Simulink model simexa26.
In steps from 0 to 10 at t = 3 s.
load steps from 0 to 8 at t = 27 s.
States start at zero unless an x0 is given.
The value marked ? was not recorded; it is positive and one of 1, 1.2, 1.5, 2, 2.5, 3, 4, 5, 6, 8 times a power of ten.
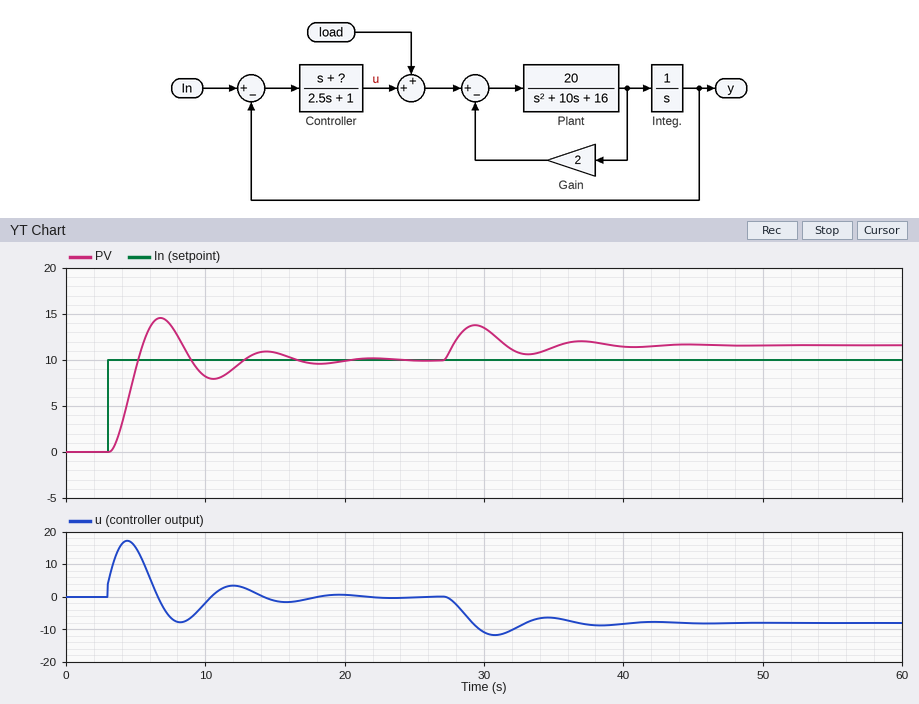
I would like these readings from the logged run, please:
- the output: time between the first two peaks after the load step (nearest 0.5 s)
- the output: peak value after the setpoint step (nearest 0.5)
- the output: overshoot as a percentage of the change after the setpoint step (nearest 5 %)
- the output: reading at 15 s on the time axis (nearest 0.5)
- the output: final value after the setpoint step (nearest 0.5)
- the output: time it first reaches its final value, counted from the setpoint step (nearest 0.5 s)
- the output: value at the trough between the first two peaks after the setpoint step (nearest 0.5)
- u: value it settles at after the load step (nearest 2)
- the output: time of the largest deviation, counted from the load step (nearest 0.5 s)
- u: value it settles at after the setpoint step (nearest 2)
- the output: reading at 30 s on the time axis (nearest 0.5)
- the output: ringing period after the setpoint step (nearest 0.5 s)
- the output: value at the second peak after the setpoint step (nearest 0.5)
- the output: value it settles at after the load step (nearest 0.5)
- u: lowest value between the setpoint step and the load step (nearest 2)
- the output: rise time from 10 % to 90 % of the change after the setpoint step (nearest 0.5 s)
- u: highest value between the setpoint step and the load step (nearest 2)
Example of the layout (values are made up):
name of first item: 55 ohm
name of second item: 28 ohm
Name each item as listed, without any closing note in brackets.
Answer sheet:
the output: time between the first two peaks after the load step: 7.5 s
the output: peak value after the setpoint step: 14.5
the output: overshoot as a percentage of the change after the setpoint step: 45 %
the output: reading at 15 s on the time axis: 11.0
the output: final value after the setpoint step: 10.0
the output: time it first reaches its final value, counted from the setpoint step: 2.0 s
the output: value at the trough between the first two peaks after the setpoint step: 8.0
u: value it settles at after the load step: -8
the output: time of the largest deviation, counted from the load step: 2.5 s
u: value it settles at after the setpoint step: 0
the output: reading at 30 s on the time axis: 13.5
the output: ringing period after the setpoint step: 7.5 s
the output: value at the second peak after the setpoint step: 11.0
the output: value it settles at after the load step: 11.5
u: lowest value between the setpoint step and the load step: -8
the output: rise time from 10 % to 90 % of the change after the setpoint step: 1.5 s
u: highest value between the setpoint step and the load step: 18
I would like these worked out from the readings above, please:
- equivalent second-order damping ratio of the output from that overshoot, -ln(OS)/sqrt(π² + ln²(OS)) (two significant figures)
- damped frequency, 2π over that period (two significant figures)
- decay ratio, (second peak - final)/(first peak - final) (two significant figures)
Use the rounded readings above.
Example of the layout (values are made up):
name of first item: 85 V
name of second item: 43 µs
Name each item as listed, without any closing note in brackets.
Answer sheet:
equivalent second-order damping ratio of the output from that overshoot, -ln(OS)/sqrt(π² + ln²(OS)): 0.25
damped frequency, 2π over that period: 0.84 rad/s
decay ratio, (second peak - final)/(first peak - final): 0.22
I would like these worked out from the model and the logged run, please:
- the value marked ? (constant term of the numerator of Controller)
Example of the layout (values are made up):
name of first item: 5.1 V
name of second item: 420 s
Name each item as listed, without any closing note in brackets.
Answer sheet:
the value marked ?: 5
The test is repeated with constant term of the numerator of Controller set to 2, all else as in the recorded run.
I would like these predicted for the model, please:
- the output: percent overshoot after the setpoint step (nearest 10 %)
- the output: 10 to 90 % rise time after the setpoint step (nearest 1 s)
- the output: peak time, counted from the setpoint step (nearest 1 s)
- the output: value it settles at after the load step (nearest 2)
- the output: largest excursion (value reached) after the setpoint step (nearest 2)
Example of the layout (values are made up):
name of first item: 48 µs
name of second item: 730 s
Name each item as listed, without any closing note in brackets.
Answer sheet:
the output: percent overshoot after the setpoint step: 20 %
the output: 10 to 90 % rise time after the setpoint step: 3 s
the output: peak time, counted from the setpoint step: 6 s
the output: value it settles at after the load step: 14
the output: largest excursion (value reached) after the setpoint step: 12
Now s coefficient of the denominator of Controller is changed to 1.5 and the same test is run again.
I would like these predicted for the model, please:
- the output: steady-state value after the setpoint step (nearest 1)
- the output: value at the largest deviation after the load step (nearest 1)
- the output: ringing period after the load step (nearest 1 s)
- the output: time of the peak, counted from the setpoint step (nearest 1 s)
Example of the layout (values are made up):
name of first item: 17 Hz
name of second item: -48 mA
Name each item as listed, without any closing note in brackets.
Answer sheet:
the output: steady-state value after the setpoint step: 10
the output: value at the largest deviation after the load step: 13
the output: ringing period after the load step: 6 s
the output: time of the peak, counted from the setpoint step: 3 s
